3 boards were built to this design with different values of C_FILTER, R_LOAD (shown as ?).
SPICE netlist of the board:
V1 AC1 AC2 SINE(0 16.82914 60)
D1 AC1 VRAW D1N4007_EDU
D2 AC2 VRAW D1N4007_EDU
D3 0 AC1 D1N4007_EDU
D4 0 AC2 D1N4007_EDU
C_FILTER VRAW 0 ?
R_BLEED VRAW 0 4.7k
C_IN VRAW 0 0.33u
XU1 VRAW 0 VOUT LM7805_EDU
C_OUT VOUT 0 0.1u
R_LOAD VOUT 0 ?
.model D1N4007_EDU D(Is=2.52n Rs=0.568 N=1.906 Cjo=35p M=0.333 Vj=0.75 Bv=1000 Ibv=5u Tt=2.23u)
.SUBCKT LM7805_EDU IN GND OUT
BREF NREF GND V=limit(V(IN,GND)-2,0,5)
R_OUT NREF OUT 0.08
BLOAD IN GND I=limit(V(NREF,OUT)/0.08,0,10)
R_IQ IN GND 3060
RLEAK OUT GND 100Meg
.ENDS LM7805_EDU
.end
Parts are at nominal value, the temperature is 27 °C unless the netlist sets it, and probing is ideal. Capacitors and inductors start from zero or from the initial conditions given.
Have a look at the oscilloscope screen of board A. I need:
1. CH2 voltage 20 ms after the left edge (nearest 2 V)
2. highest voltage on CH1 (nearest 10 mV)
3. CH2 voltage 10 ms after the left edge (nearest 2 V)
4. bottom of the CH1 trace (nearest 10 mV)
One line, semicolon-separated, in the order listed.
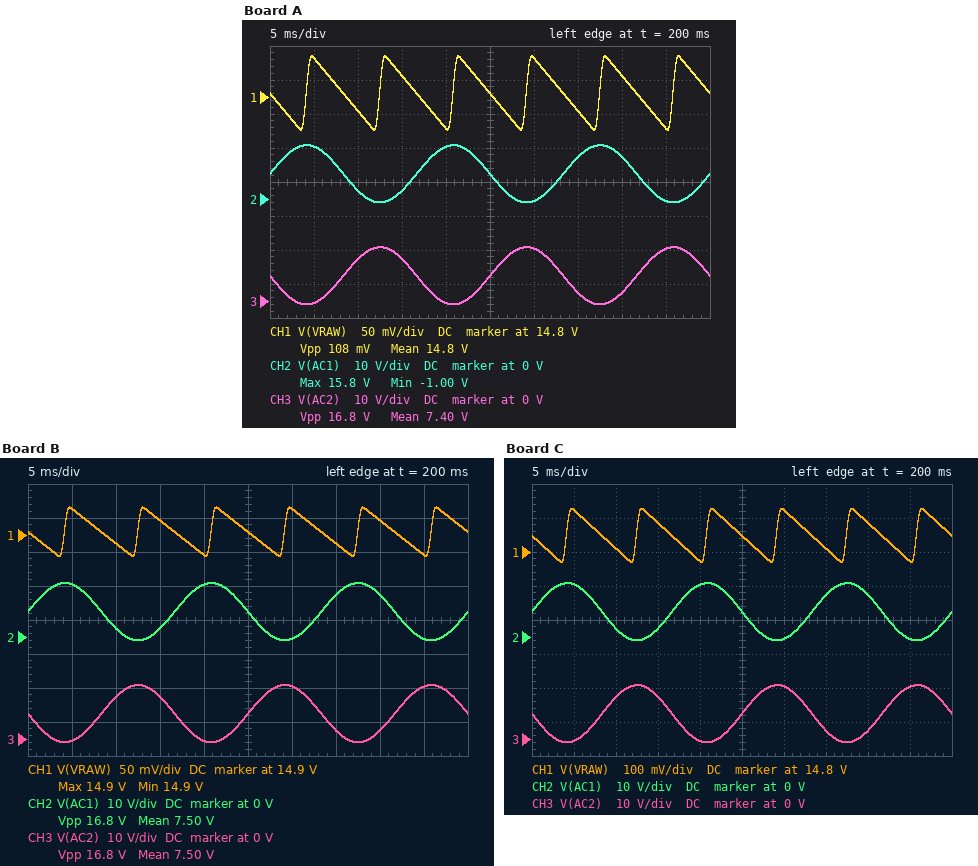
16 V; 14.86 V; 2 V; 14.75 V
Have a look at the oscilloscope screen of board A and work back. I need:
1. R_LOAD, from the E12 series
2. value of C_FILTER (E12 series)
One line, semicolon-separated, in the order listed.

470 Ω; 1.2 mF
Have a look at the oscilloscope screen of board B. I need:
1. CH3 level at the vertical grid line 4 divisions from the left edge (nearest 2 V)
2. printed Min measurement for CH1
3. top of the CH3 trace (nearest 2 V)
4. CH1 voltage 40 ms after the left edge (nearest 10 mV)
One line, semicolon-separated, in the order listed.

0 V; 14.9 V; 16 V; 14.92 V
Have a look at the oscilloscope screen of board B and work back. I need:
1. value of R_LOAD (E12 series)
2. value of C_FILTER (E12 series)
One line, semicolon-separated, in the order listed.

1.2 kΩ; 1.2 mF
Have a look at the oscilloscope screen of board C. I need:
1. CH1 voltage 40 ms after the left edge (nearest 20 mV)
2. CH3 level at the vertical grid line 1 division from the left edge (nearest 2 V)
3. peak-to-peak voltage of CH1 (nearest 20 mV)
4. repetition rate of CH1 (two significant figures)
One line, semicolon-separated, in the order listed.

14.88 V; 0 V; 160 mV; 120 Hz
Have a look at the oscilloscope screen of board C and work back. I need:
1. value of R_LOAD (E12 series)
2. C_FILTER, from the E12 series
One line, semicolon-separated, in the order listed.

680 Ω; 680 µF
